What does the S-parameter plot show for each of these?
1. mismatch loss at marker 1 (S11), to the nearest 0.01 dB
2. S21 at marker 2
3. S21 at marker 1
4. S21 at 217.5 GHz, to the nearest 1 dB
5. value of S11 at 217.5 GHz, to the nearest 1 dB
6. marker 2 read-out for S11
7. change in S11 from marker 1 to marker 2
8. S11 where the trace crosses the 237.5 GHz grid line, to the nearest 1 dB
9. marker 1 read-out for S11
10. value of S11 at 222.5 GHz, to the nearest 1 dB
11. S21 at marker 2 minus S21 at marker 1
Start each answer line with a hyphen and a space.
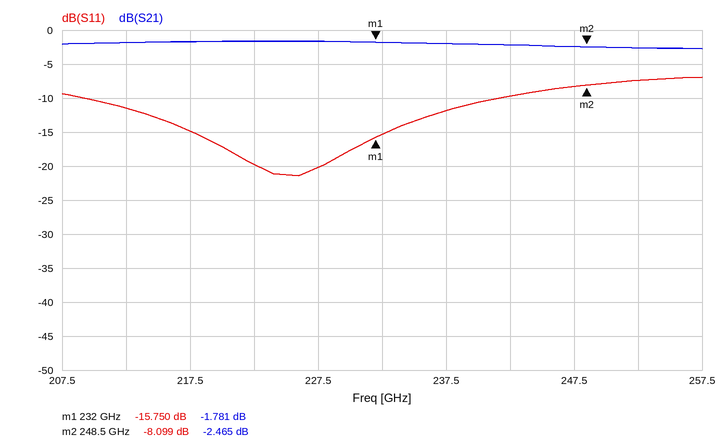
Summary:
- 0.12 dB
- -2.465 dB
- -1.781 dB
- -2 dB
- -15 dB
- -8.099 dB
- 7.651 dB
- -12 dB
- -15.750 dB
- -20 dB
- -0.684 dB
